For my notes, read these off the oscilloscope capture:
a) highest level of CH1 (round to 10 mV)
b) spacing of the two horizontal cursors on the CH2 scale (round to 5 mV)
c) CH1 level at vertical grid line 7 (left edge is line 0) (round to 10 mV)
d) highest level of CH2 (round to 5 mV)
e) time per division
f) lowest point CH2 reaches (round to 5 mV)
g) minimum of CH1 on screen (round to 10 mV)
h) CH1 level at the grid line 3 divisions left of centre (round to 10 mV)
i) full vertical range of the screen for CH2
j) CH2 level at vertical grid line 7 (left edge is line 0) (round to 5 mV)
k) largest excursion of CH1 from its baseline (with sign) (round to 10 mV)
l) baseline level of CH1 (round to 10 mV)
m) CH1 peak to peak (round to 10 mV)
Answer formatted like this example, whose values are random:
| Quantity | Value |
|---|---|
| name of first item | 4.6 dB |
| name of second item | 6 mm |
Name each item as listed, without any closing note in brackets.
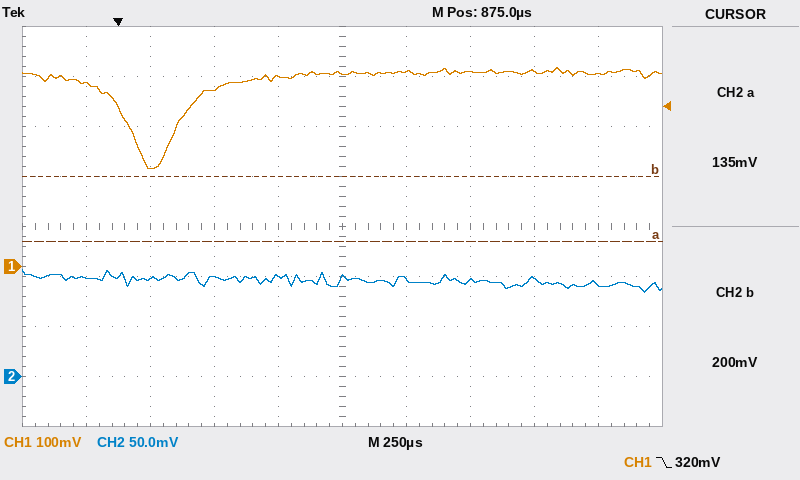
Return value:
| Quantity | Value |
|---|---|
| highest level of CH1 | 400 mV |
| spacing of the two horizontal cursors on the CH2 scale | 65 mV |
| CH1 level at vertical grid line 7 (left edge is line 0) | 390 mV |
| highest level of CH2 | 105 mV |
| time per division | 250 µs |
| lowest point CH2 reaches | 85 mV |
| minimum of CH1 on screen | 200 mV |
| CH1 level at the grid line 3 divisions left of centre | 200 mV |
| full vertical range of the screen for CH2 | 400 mV |
| CH2 level at vertical grid line 7 (left edge is line 0) | 95 mV |
| largest excursion of CH1 from its baseline (with sign) | -190 mV |
| baseline level of CH1 | 390 mV |
| CH1 peak to peak | 200 mV |
